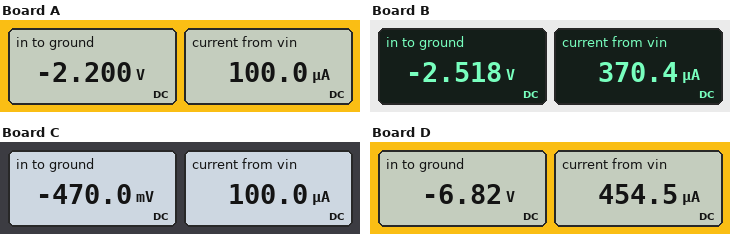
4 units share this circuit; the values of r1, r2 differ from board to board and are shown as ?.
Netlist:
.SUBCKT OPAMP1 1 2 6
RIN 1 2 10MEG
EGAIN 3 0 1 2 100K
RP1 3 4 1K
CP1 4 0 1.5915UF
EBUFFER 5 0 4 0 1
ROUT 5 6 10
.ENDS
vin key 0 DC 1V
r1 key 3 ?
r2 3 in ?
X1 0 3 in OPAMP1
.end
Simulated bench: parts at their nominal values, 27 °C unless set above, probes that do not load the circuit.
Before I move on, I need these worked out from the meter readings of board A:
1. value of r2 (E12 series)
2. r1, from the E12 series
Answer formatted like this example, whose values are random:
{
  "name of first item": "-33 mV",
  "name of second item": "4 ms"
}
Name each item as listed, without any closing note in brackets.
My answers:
{
  "value of r2": "22 kΩ",
  "r1, from the E12 series": "10 kΩ"
}
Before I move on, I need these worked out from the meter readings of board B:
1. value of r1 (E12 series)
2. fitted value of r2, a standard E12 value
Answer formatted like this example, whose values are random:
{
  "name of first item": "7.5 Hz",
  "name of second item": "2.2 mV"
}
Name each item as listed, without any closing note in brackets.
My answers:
{
  "value of r1": "2.7 kΩ",
  "fitted value of r2, a standard E12 value": "6.8 kΩ"
}
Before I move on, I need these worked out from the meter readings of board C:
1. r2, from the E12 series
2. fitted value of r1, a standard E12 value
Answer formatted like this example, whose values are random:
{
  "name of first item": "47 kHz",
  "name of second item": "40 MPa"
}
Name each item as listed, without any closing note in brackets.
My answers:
{
  "r2, from the E12 series": "4.7 kΩ",
  "fitted value of r1, a standard E12 value": "10 kΩ"
}
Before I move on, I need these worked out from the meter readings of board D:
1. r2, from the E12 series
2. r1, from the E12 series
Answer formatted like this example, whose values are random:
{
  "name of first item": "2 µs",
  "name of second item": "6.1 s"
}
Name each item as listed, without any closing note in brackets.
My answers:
{
  "r2, from the E12 series": "15 kΩ",
  "r1, from the E12 series": "2.2 kΩ"
}
